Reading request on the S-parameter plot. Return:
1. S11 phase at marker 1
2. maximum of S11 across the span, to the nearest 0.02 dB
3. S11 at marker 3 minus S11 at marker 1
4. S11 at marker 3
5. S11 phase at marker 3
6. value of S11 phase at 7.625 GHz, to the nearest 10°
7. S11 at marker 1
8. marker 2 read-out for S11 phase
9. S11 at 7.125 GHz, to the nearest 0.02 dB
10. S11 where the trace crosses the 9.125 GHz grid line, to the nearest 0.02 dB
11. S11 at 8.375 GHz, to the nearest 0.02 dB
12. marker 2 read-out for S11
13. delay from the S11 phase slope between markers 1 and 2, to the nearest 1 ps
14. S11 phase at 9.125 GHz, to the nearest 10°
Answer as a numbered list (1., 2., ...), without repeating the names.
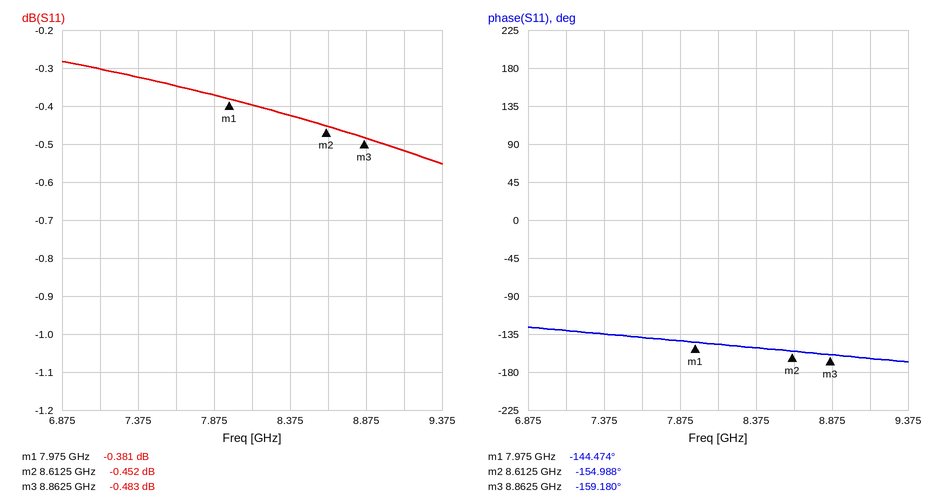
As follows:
1. -144.474°
2. -0.28 dB
3. -0.102 dB
4. -0.483 dB
5. -159.180°
6. -140°
7. -0.381 dB
8. -154.988°
9. -0.30 dB
10. -0.52 dB
11. -0.42 dB
12. -0.452 dB
13. 46 ps
14. -160°
